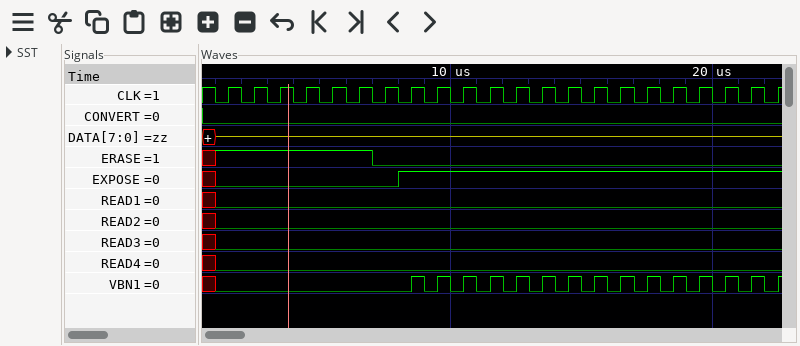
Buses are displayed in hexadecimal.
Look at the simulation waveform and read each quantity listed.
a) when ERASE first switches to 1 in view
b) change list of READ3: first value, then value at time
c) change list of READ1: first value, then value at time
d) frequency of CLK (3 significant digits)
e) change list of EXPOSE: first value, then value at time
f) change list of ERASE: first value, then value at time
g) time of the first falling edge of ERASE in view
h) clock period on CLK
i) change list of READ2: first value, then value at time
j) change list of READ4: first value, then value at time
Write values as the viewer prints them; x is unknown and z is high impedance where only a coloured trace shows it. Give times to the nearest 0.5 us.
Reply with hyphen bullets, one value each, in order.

- 1 us
- x, 0 at 1 us
- x, 0 at 1 us
- 1.00 MHz
- x, 0 at 1 us, 1 at 8 us
- x, 1 at 1 us, 0 at 7 us
- 7 us
- 1 us
- x, 0 at 1 us
- x, 0 at 1 us
